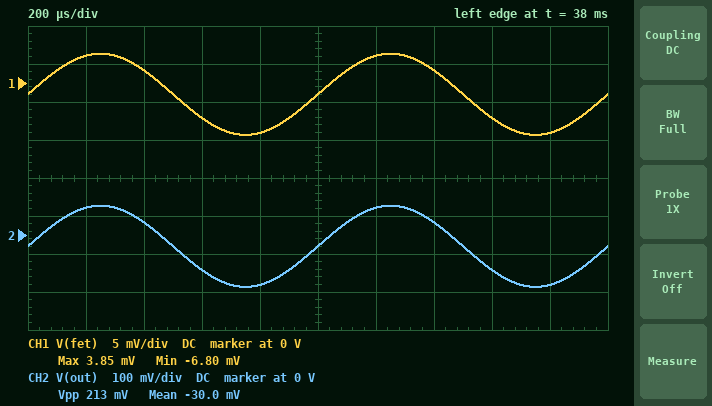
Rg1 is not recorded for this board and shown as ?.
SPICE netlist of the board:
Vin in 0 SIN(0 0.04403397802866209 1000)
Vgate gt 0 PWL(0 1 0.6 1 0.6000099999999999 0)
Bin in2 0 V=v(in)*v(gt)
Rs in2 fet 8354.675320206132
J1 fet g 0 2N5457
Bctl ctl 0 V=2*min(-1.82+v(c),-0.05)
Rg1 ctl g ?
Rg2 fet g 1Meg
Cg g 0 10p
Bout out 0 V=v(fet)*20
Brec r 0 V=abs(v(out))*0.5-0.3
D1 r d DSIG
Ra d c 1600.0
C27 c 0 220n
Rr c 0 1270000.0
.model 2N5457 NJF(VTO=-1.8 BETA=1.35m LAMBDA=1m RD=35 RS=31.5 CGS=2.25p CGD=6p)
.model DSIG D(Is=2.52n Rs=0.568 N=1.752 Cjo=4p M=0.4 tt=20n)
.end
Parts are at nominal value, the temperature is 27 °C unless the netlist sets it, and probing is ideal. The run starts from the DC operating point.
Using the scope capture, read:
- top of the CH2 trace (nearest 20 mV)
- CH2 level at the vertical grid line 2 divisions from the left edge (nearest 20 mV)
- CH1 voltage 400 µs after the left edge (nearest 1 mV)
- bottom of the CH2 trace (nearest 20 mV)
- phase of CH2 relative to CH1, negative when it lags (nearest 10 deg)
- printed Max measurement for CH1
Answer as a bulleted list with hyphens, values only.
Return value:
- 80 mV
- 40 mV
- 2 mV
- -140 mV
- 0 deg
- 3.85 mV
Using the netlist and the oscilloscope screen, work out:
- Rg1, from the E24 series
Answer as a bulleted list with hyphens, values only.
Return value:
- 1.5 MΩ
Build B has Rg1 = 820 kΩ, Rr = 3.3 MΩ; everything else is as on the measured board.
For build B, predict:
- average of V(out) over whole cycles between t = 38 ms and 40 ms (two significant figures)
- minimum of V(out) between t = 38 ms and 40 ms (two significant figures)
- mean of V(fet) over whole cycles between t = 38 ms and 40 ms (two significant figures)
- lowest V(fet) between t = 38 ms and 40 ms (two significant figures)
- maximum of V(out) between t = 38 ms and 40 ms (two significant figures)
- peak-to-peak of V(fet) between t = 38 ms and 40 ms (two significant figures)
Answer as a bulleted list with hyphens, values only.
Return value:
- -330 mV
- -1.2 V
- -16 mV
- -60 mV
- 550 mV
- 88 mV
